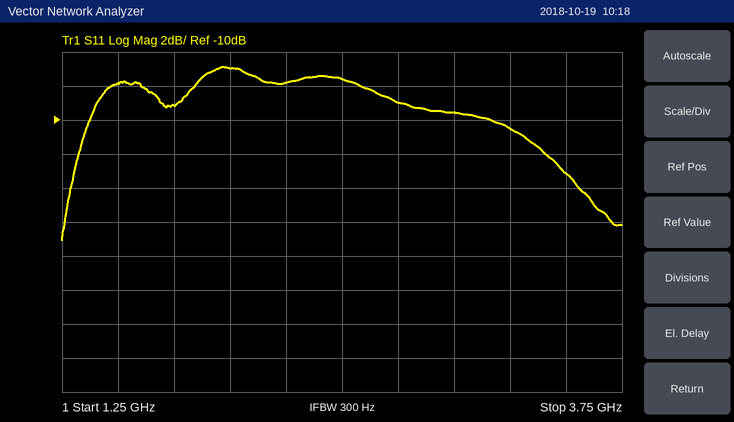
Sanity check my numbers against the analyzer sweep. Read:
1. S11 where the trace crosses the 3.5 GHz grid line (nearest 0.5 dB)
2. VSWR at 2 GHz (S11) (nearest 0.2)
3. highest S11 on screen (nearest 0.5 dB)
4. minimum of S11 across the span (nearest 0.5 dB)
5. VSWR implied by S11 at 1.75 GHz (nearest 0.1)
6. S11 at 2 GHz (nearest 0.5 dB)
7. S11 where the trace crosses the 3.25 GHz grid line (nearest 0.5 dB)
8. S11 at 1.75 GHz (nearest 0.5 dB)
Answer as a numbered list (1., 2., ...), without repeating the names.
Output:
1. -13.0 dB
2. 2.6
3. -7.0 dB
4. -17.0 dB
5. 2.1
6. -7.0 dB
7. -10.5 dB
8. -9.0 dB
